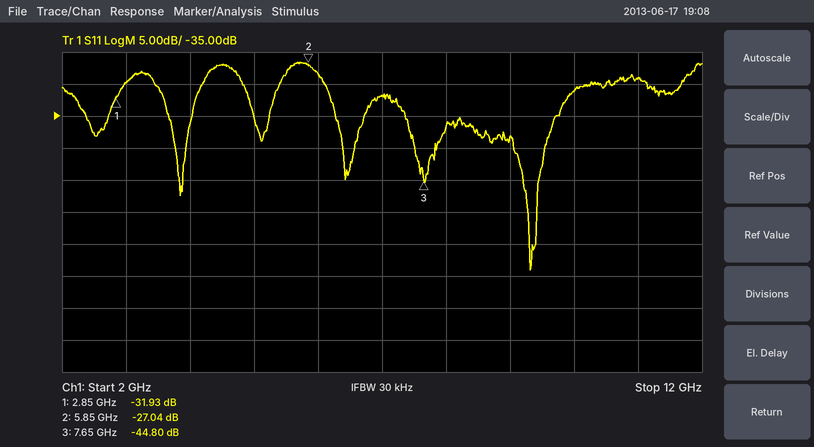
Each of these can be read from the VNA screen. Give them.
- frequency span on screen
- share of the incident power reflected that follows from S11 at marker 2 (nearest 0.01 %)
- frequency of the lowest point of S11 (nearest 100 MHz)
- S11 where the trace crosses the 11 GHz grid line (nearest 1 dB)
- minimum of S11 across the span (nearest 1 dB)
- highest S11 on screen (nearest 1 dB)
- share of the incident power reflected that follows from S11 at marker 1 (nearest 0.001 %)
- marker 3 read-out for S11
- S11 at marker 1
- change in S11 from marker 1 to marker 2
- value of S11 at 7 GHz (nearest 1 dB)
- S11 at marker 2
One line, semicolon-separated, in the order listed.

10 GHz; 0.20 %; 9.3 GHz; -29 dB; -59 dB; -27 dB; 0.064 %; -44.80 dB; -31.93 dB; 4.89 dB; -32 dB; -27.04 dB
